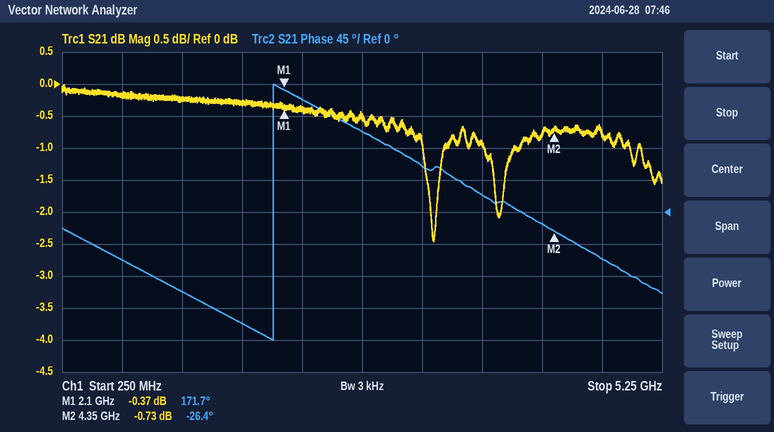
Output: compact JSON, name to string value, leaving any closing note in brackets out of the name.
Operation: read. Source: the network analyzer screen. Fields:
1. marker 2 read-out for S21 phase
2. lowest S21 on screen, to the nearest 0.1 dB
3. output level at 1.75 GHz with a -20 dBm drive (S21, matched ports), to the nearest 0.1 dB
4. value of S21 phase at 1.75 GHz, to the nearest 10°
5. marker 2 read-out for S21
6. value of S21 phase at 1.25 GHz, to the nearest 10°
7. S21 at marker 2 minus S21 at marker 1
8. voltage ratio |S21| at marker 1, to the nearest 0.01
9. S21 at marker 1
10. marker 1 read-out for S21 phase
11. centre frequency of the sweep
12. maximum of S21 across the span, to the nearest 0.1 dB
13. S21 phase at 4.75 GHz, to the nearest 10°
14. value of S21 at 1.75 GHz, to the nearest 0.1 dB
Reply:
{"marker 2 read-out for S21 phase": "-26.4°", "lowest S21 on screen, to the nearest 0.1 dB": "-2.5 dB", "output level at 1.75 GHz with a -20 dBm drive (S21, matched ports), to the nearest 0.1 dB": "-20.3 dBm", "value of S21 phase at 1.75 GHz, to the nearest 10°": "-160°", "marker 2 read-out for S21": "-0.73 dB", "value of S21 phase at 1.25 GHz, to the nearest 10°": "-110°", "S21 at marker 2 minus S21 at marker 1": "-0.36 dB", "voltage ratio |S21| at marker 1, to the nearest 0.01": "0.96", "S21 at marker 1": "-0.37 dB", "marker 1 read-out for S21 phase": "171.7°", "centre frequency of the sweep": "2.75 GHz", "maximum of S21 across the span, to the nearest 0.1 dB": "0.0 dB", "S21 phase at 4.75 GHz, to the nearest 10°": "-70°", "value of S21 at 1.75 GHz, to the nearest 0.1 dB": "-0.3 dB"}
